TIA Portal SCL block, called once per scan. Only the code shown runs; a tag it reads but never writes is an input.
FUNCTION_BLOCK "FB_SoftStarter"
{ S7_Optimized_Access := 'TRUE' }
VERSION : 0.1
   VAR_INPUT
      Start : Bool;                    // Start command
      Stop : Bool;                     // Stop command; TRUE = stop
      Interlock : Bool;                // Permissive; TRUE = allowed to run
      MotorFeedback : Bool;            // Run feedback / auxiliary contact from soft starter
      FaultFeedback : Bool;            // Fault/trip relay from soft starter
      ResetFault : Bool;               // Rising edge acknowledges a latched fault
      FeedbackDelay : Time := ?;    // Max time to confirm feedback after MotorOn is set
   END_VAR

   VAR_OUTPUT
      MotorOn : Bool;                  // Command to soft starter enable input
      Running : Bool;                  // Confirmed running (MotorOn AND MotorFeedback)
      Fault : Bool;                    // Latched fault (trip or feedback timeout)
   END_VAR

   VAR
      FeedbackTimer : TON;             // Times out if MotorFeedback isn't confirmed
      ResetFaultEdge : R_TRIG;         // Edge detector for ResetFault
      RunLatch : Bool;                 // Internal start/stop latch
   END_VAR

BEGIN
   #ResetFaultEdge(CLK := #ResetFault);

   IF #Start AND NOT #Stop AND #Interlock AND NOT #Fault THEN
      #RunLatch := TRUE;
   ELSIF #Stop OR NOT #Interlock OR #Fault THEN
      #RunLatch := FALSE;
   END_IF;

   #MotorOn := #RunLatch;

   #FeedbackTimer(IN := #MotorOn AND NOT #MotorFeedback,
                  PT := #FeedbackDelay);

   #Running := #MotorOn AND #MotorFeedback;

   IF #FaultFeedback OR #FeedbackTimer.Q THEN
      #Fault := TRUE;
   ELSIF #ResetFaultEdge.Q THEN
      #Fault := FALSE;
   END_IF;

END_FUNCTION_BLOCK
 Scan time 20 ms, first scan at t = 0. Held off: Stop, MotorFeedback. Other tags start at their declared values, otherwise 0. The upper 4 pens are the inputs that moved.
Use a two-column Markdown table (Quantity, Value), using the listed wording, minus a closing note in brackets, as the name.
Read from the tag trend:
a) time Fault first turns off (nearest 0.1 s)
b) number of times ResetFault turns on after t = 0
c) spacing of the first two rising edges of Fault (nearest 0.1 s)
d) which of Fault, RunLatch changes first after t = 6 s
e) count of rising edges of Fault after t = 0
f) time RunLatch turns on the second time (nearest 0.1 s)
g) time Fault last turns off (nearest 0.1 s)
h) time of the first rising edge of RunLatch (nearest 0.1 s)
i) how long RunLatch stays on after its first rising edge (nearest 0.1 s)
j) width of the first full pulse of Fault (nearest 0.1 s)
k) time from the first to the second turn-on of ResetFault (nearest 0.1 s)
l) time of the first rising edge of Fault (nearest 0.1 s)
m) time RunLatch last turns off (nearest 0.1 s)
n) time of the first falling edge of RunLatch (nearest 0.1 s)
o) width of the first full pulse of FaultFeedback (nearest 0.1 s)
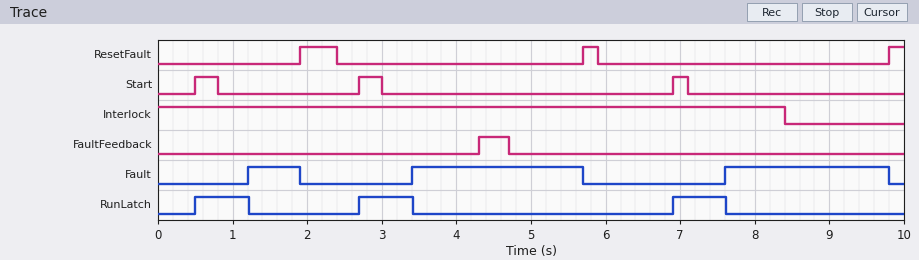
| Quantity | Value |
|---|---|
| time Fault first turns off | 1.9 s |
| number of times ResetFault turns on after t = 0 | 3 |
| spacing of the first two rising edges of Fault | 2.2 s |
| which of Fault, RunLatch changes first after t = 6 s | RunLatch |
| count of rising edges of Fault after t = 0 | 3 |
| time RunLatch turns on the second time | 2.7 s |
| time Fault last turns off | 9.8 s |
| time of the first rising edge of RunLatch | 0.5 s |
| how long RunLatch stays on after its first rising edge | 0.7 s |
| width of the first full pulse of Fault | 0.7 s |
| time from the first to the second turn-on of ResetFault | 3.8 s |
| time of the first rising edge of Fault | 1.2 s |
| time RunLatch last turns off | 7.6 s |
| time of the first falling edge of RunLatch | 1.2 s |
| width of the first full pulse of FaultFeedback | 0.4 s |
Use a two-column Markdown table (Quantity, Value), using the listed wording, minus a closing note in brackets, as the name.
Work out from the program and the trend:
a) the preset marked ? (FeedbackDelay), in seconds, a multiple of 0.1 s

| Quantity | Value |
|---|---|
| the preset marked ? (FeedbackDelay), in seconds, a multiple of 0.1 s | 0.7 s |
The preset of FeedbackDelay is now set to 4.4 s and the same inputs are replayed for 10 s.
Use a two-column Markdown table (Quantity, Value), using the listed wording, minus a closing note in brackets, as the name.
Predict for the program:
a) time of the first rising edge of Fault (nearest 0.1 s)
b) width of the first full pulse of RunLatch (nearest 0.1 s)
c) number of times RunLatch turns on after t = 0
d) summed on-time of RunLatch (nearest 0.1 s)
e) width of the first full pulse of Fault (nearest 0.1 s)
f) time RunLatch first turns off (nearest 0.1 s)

| Quantity | Value |
|---|---|
| time of the first rising edge of Fault | 4.3 s |
| width of the first full pulse of RunLatch | 3.8 s |
| number of times RunLatch turns on after t = 0 | 2 |
| summed on-time of RunLatch | 5.3 s |
| width of the first full pulse of Fault | 1.4 s |
| time RunLatch first turns off | 4.3 s |
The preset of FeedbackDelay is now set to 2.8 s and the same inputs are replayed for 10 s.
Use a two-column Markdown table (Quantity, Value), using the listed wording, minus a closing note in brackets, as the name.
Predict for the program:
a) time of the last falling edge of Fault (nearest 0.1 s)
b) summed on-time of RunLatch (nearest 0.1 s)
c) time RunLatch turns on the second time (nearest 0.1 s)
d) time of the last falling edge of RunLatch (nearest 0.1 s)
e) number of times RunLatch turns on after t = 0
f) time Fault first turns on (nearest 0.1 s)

| Quantity | Value |
|---|---|
| time of the last falling edge of Fault | 5.7 s |
| summed on-time of RunLatch | 4.3 s |
| time RunLatch turns on the second time | 6.9 s |
| time of the last falling edge of RunLatch | 8.4 s |
| number of times RunLatch turns on after t = 0 | 2 |
| time Fault first turns on | 3.3 s |
